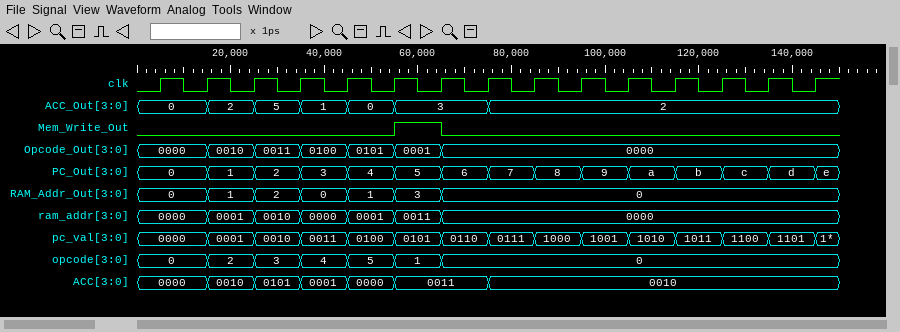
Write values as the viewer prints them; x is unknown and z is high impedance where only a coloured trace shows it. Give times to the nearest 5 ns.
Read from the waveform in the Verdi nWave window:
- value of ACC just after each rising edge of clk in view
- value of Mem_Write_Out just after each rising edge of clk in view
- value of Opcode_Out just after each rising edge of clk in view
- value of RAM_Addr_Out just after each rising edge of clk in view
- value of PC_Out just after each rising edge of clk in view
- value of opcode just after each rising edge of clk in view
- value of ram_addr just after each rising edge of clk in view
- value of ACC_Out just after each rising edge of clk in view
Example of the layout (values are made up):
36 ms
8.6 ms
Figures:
0000, 0010, 0101, 0001, 0000, 0011, 0011, 0010, 0010, 0010, 0010, 0010, 0010, 0010, 0010
0 0 0 0 0 1 0 0 0 0 0 0 0 0 0
0000, 0010, 0011, 0100, 0101, 0001, 0000, 0000, 0000, 0000, 0000, 0000, 0000, 0000, 0000
0, 1, 2, 0, 1, 3, 0, 0, 0, 0, 0, 0, 0, 0, 0
0, 1, 2, 3, 4, 5, 6, 7, 8, 9, a, b, c, d, e
0, 2, 3, 4, 5, 1, 0, 0, 0, 0, 0, 0, 0, 0, 0
0000, 0001, 0010, 0000, 0001, 0011, 0000, 0000, 0000, 0000, 0000, 0000, 0000, 0000, 0000
0, 2, 5, 1, 0, 3, 3, 2, 2, 2, 2, 2, 2, 2, 2
